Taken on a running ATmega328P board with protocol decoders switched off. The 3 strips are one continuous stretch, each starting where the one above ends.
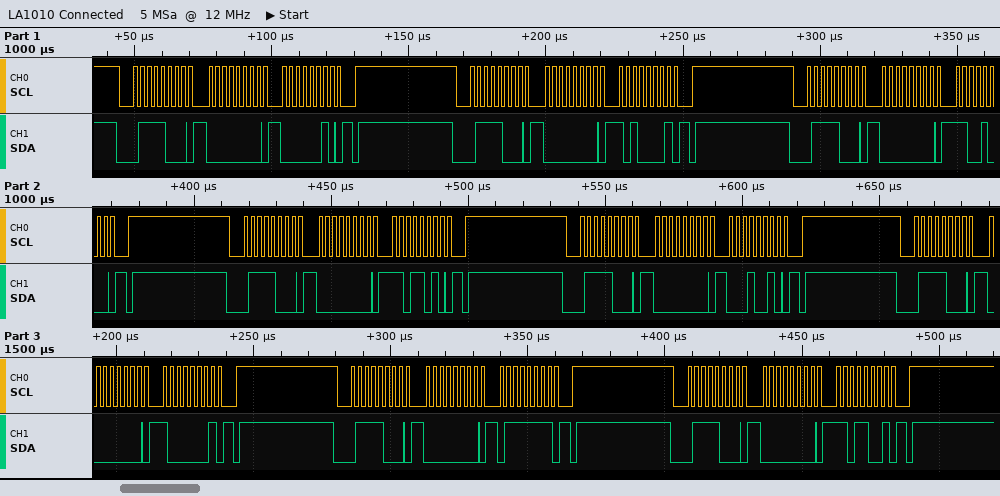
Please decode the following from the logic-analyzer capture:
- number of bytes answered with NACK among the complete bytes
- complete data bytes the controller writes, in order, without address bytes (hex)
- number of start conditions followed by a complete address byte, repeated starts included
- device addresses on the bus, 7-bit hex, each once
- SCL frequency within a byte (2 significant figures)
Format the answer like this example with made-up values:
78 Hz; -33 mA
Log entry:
0; 00 02 00 A1 00 C8 00 DA 00 12 00 81 00 7F 00 D9; 8; 0x3C; 400 kHz
